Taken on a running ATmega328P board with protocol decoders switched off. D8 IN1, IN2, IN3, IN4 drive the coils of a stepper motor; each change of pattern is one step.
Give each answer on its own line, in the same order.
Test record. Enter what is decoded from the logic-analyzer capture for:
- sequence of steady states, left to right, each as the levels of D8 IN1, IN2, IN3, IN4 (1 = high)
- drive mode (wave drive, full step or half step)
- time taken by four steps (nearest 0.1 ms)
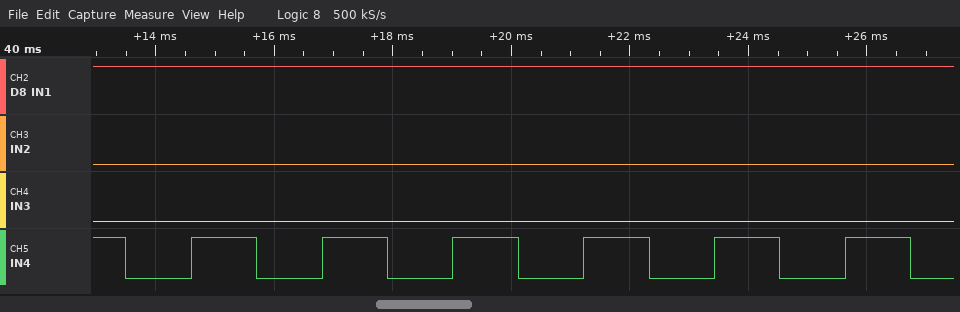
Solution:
1001 1000 1001 1000 1001 1000 1001 1000 1001 1000 1001 1000 1001 1000
half step
4.4 ms
